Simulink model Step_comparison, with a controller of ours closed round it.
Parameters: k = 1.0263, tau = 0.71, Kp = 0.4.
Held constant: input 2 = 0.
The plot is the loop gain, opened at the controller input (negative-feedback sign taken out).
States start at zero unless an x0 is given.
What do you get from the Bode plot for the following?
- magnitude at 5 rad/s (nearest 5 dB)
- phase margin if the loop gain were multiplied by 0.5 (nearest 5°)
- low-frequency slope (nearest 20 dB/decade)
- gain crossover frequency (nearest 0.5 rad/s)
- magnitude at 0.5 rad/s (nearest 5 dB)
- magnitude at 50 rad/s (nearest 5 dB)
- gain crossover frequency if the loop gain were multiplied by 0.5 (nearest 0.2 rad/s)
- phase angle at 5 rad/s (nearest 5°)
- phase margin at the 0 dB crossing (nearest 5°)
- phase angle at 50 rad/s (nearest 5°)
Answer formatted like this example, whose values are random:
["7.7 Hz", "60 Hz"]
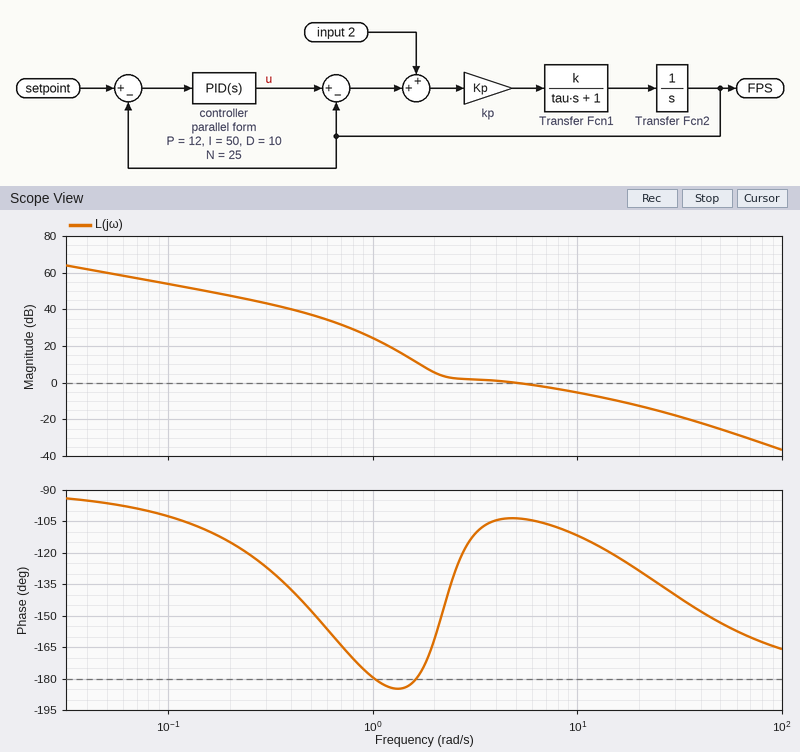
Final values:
["0 dB", "15°", "-20 dB/decade", "5.0 rad/s", "35 dB", "-25 dB", "2.0 rad/s", "-105°", "75°", "-155°"]
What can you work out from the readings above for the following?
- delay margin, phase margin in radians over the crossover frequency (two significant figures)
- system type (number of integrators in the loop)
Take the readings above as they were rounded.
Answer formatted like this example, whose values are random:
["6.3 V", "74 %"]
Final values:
["0.26 s", "1"]
